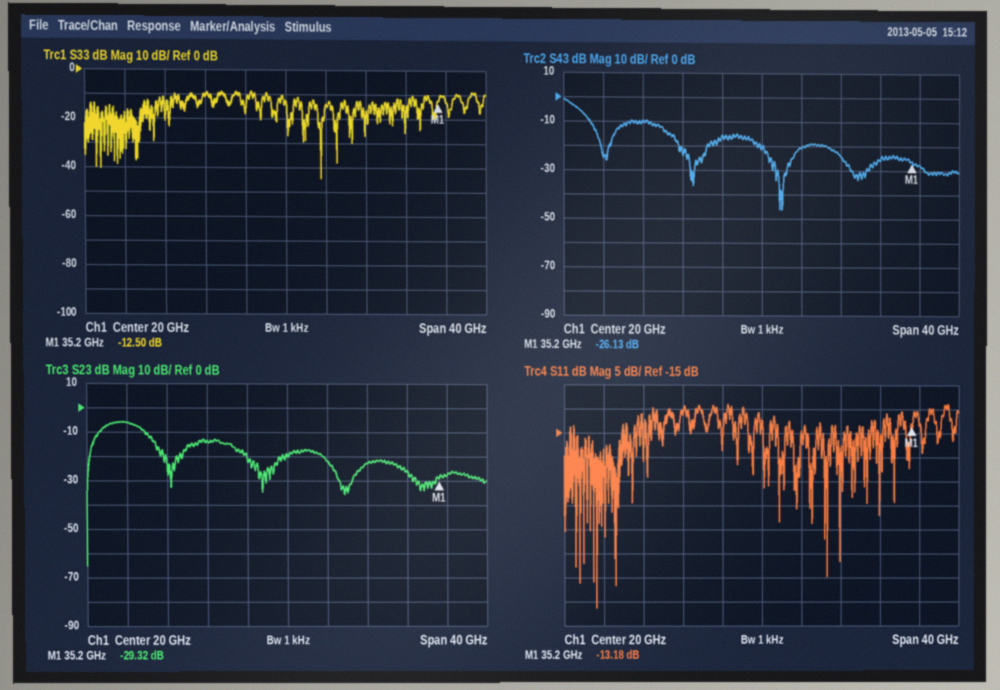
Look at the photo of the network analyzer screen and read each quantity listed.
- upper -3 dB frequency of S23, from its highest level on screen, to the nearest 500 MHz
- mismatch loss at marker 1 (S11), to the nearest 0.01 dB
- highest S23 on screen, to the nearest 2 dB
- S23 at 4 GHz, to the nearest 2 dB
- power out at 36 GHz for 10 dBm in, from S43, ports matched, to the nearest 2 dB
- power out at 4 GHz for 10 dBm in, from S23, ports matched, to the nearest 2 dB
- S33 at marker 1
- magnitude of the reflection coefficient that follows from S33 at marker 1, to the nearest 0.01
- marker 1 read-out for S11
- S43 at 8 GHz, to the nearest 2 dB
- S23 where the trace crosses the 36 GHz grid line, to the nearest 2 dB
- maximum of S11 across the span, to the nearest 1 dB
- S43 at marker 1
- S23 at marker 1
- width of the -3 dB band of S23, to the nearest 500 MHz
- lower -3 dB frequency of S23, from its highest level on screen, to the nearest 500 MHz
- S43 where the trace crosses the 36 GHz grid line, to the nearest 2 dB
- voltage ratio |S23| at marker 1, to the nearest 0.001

5.5 GHz
0.21 dB
-6 dB
-6 dB
-18 dBm
4 dBm
-12.50 dB
0.24
-13.18 dB
-10 dB
-28 dB
-9 dB
-26.13 dB
-29.32 dB
4.0 GHz
1.5 GHz
-28 dB
0.034
